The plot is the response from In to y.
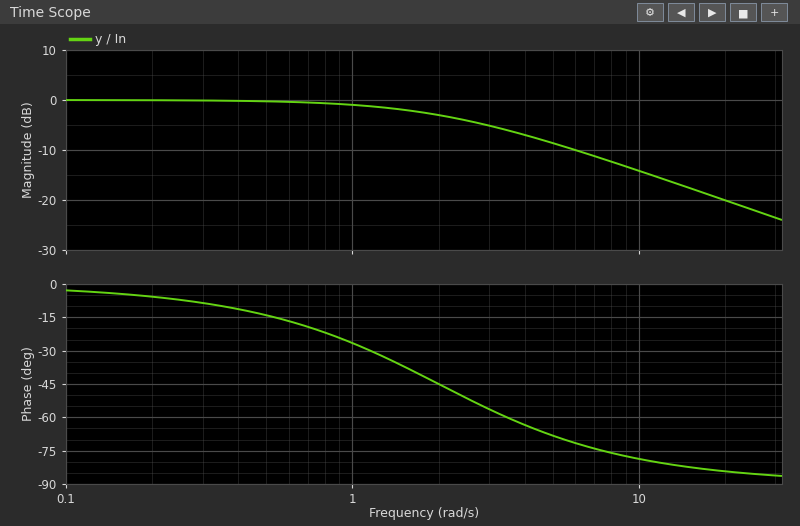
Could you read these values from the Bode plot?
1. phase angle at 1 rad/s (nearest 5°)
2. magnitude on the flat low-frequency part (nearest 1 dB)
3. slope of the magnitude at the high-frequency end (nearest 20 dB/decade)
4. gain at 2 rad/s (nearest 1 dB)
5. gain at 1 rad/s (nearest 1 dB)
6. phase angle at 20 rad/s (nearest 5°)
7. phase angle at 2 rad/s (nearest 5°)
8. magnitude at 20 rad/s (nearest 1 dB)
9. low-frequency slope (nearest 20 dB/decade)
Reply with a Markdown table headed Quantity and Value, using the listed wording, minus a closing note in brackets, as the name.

| Quantity | Value |
|---|---|
| phase angle at 1 rad/s | -25° |
| magnitude on the flat low-frequency part | 0 dB |
| slope of the magnitude at the high-frequency end | -20 dB/decade |
| gain at 2 rad/s | -3 dB |
| gain at 1 rad/s | -1 dB |
| phase angle at 20 rad/s | -85° |
| phase angle at 2 rad/s | -45° |
| magnitude at 20 rad/s | -20 dB |
| low-frequency slope | 0 dB/decade |
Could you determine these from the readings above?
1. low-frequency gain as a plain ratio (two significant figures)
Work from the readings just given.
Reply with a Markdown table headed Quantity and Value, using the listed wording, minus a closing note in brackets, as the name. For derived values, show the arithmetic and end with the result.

| Quantity | Value |
|---|---|
| low-frequency gain as a plain ratio | 10^(0 / 20) = 1.0 |
